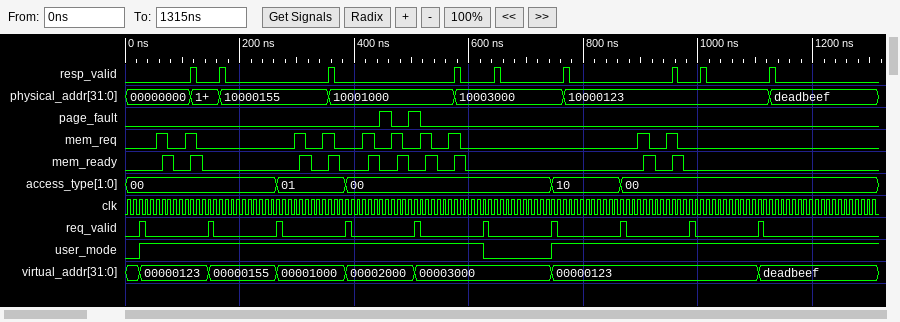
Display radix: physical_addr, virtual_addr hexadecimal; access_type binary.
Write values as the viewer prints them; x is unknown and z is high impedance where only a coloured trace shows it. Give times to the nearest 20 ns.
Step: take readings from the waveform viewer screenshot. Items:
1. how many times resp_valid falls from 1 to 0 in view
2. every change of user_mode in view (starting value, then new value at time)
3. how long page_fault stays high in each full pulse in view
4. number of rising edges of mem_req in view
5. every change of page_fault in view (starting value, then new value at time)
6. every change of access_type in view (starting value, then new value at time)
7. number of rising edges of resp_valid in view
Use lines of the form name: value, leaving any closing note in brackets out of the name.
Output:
how many times resp_valid falls from 1 to 0 in view: 9
every change of user_mode in view: 0, 1 at 20 ns, 0 at 620 ns, 1 at 740 ns
how long page_fault stays high in each full pulse in view: 20 ns, 20 ns
number of rising edges of mem_req in view: 10
every change of page_fault in view: 0, 1 at 440 ns, 0 at 460 ns, 1 at 500 ns, 0 at 520 ns
every change of access_type in view: 00, 01 at 260 ns, 00 at 380 ns, 10 at 740 ns, 00 at 860 ns
number of rising edges of resp_valid in view: 9
